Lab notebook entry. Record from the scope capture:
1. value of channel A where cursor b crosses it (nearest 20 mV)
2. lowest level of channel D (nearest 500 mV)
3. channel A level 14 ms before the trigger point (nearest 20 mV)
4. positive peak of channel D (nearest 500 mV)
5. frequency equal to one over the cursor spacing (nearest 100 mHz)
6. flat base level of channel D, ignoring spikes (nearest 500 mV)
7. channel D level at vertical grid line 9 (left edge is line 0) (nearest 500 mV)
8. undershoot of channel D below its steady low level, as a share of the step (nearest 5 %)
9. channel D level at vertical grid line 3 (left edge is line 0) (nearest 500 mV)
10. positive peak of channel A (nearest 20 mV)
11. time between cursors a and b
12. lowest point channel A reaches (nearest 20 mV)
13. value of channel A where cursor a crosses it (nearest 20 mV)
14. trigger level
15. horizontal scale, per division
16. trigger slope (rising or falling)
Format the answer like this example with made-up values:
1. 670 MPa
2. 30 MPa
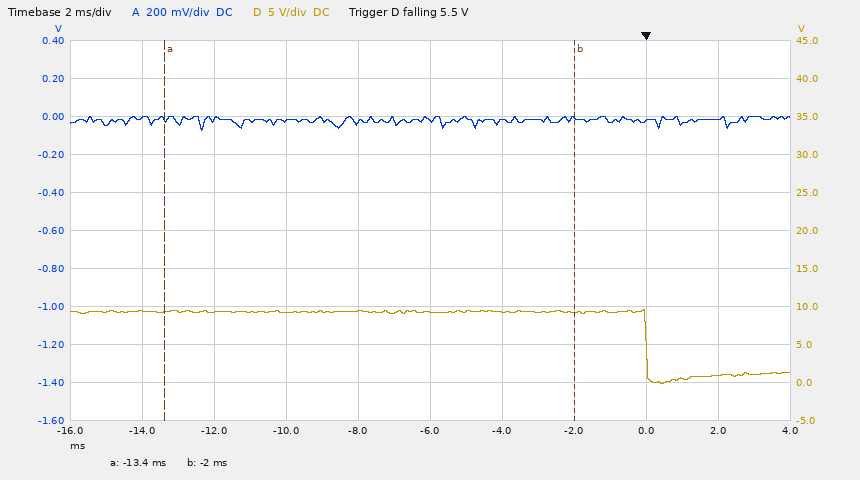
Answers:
1. 0 mV
2. 0.0 V
3. 0 mV
4. 9.5 V
5. 87.7 Hz
6. 1.0 V
7. 1.0 V
8. 15 %
9. 9.0 V
10. 0 mV
11. 11.4 ms
12. -80 mV
13. -20 mV
14. 5.5 V
15. 2 ms
16. falling
